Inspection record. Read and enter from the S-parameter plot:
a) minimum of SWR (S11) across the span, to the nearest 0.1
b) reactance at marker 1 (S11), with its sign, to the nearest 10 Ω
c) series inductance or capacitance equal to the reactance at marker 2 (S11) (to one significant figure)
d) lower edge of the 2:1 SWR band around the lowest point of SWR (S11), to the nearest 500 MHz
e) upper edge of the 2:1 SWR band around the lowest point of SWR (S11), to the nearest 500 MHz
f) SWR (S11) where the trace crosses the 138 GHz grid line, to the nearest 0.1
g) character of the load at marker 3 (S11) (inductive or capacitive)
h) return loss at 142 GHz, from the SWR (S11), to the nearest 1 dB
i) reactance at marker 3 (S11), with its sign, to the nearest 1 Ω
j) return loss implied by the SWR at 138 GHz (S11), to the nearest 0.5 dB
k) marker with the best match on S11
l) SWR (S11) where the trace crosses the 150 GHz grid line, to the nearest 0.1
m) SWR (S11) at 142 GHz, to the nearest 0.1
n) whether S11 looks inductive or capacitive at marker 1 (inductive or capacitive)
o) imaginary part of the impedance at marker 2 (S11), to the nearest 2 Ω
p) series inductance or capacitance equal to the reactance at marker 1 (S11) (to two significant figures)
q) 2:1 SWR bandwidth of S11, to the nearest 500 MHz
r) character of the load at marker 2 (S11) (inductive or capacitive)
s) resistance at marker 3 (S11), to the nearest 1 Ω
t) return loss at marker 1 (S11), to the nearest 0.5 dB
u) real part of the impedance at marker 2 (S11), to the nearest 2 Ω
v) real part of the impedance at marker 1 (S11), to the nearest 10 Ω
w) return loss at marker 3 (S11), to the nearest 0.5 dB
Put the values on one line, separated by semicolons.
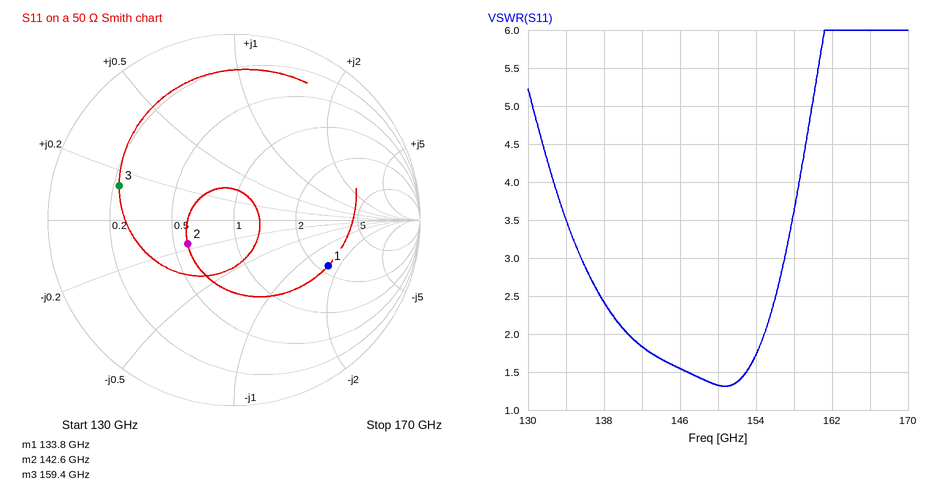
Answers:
1.3; -80 Ω; 100 fF; 140.5 GHz; 155.0 GHz; 2.4; inductive; 11 dB; +7 Ω; 7.5 dB; marker 2; 1.3; 1.8; capacitive; -8 Ω; 15 fF; 14.5 GHz; capacitive; 11 Ω; 5.0 dB; 30 Ω; 110 Ω; 4.0 dB
